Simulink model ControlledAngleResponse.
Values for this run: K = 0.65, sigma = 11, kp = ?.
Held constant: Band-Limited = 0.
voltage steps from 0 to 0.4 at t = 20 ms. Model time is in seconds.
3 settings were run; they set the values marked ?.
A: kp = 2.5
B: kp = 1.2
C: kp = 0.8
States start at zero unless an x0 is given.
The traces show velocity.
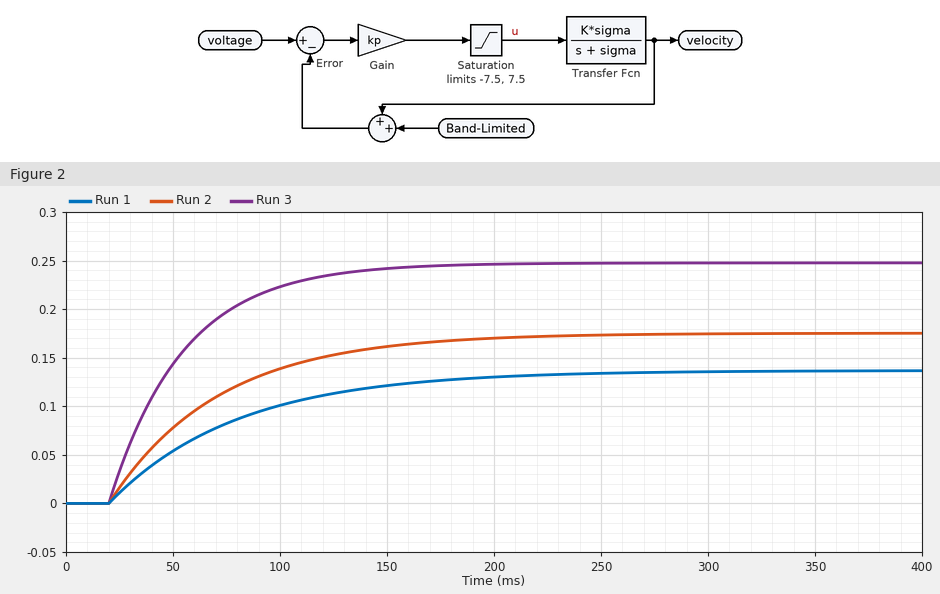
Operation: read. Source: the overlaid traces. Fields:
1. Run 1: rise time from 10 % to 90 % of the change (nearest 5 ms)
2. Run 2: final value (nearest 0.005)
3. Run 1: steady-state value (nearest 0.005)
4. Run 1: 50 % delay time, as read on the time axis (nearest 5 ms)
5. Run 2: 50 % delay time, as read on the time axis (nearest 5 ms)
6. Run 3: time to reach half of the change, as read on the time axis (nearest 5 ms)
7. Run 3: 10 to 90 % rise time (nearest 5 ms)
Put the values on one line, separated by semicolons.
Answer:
130 ms; 0.175; 0.135; 60 ms; 55 ms; 45 ms; 75 ms
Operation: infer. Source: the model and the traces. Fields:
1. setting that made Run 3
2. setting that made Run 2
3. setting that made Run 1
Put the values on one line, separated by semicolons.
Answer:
A; B; C
